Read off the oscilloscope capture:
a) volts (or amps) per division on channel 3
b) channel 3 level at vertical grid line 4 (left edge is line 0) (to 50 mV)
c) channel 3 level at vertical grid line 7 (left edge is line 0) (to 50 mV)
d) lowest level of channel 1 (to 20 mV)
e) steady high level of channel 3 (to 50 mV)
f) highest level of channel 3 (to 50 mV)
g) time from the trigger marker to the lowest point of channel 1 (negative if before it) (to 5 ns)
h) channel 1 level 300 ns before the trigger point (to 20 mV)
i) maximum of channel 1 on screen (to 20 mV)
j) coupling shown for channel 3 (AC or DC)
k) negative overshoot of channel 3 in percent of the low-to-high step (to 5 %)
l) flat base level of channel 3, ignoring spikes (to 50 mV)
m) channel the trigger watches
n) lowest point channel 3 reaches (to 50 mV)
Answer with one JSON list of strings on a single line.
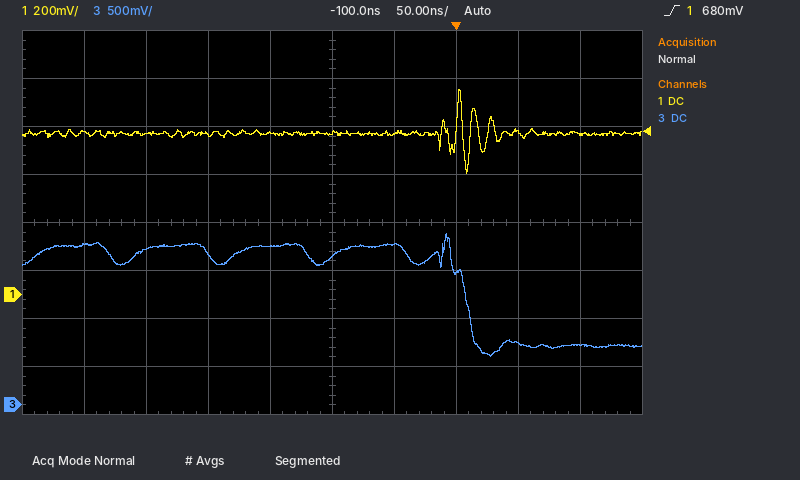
["500 mV", "1.65 V", "1.40 V", "500 mV", "1.65 V", "1.80 V", "+10 ns", "680 mV", "860 mV", "DC", "10 %", "600 mV", "channel 1", "500 mV"]
